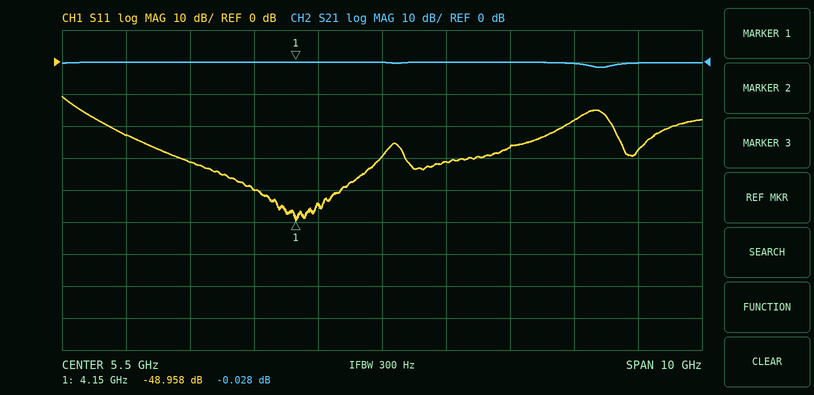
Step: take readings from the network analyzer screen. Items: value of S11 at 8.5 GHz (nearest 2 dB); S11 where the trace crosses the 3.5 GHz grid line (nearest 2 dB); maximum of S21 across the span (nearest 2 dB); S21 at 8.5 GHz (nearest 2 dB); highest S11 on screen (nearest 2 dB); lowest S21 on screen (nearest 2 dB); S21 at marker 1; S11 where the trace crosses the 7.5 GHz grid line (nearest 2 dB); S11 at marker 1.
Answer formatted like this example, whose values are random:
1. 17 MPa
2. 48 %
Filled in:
1. -18 dB
2. -40 dB
3. 0 dB
4. 0 dB
5. -10 dB
6. -2 dB
7. -0.028 dB
8. -26 dB
9. -48.958 dB
